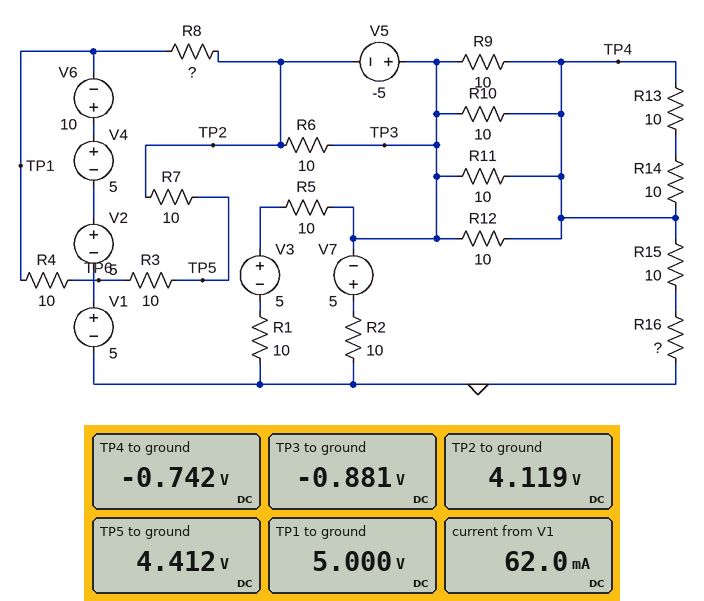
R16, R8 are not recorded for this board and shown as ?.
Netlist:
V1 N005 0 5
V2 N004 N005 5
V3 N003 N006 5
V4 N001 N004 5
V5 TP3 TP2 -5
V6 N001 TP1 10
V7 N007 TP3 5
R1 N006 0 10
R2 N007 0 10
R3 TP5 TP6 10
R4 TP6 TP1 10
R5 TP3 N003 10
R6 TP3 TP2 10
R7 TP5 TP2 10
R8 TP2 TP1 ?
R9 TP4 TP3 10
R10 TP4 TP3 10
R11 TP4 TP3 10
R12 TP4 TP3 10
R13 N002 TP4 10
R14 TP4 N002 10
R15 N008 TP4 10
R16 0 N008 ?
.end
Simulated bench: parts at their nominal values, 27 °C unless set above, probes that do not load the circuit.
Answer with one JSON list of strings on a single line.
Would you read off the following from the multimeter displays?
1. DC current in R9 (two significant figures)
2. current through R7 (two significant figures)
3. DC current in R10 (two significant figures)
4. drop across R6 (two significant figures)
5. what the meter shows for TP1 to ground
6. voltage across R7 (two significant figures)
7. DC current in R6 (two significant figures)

["14 mA", "29 mA", "14 mA", "5.0 V", "5.000 V", "290 mV", "500 mA"]
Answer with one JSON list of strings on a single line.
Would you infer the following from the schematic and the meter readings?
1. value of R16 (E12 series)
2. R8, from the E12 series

["3.3 Ω", "27 Ω"]
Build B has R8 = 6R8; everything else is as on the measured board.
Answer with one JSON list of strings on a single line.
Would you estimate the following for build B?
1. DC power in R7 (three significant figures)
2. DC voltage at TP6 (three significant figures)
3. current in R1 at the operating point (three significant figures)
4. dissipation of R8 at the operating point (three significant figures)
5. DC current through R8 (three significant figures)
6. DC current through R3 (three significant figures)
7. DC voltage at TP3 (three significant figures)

["4.48 mW", "4.79 V", "282 mA", "59.3 mW", "93.4 mA", "21.2 mA", "-635 mV"]
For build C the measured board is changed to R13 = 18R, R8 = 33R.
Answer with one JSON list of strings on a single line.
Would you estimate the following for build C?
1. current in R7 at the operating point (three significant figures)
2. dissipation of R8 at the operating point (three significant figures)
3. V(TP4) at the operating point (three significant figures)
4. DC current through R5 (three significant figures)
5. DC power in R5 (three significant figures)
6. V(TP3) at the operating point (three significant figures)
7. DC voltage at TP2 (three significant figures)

["30.1 mA", "24.7 mW", "-760 mV", "295 mA", "871 mW", "-903 mV", "4.10 V"]
